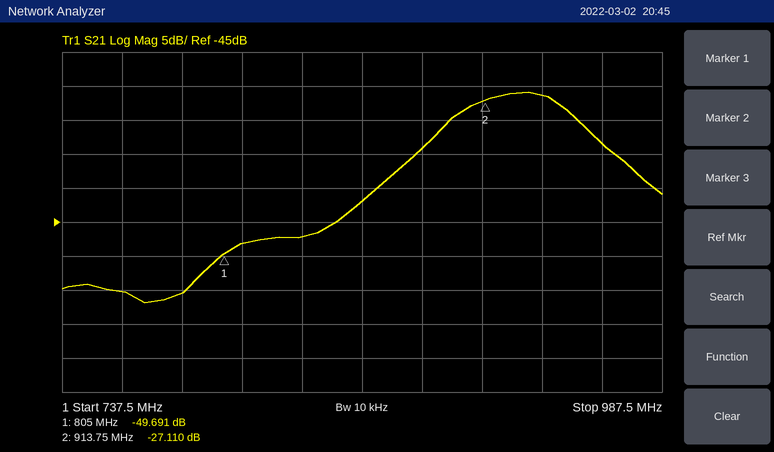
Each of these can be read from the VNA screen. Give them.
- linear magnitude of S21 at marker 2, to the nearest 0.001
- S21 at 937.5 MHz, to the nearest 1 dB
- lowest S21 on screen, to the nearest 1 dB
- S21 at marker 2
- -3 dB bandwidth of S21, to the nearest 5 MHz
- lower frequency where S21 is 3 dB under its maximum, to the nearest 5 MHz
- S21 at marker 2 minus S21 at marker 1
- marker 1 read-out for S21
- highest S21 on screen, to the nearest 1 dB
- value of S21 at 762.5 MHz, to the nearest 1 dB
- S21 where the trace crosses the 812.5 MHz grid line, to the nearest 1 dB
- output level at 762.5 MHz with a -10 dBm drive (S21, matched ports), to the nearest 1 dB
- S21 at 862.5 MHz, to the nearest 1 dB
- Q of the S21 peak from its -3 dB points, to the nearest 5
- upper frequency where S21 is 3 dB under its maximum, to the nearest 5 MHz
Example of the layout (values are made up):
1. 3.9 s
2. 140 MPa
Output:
1. 0.044
2. -26 dB
3. -57 dB
4. -27.110 dB
5. 45 MHz
6. 905 MHz
7. 22.581 dB
8. -49.691 dB
9. -26 dB
10. -55 dB
11. -48 dB
12. -65 dBm
13. -42 dB
14. 20
15. 950 MHz
